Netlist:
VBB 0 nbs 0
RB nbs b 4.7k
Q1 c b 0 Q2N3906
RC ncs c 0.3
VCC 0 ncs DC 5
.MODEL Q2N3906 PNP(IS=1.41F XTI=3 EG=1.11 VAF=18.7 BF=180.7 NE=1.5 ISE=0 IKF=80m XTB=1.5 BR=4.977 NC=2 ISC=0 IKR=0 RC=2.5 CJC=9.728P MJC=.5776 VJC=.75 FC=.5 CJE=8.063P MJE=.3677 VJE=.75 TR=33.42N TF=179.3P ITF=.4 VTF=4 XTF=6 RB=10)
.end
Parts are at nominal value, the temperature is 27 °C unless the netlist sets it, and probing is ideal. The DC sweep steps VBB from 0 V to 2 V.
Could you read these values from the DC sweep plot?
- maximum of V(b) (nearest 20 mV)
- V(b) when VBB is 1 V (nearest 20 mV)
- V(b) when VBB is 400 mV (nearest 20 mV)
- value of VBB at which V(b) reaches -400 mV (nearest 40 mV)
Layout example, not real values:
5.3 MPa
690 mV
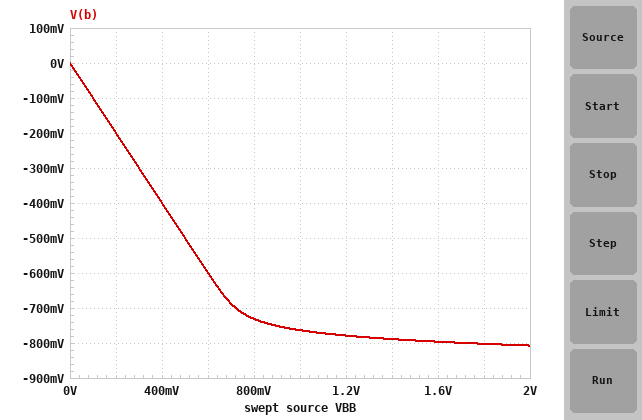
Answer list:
0 V
-760 mV
-400 mV
400 mV
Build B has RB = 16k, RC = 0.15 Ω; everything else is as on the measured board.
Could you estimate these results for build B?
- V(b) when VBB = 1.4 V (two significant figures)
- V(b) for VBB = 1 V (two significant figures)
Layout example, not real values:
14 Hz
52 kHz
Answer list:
-760 mV
-730 mV
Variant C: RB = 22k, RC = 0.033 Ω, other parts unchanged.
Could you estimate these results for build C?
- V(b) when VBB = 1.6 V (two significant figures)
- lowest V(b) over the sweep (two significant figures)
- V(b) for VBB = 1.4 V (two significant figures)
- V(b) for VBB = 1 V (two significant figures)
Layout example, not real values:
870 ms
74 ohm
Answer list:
-760 mV
-770 mV
-750 mV
-730 mV
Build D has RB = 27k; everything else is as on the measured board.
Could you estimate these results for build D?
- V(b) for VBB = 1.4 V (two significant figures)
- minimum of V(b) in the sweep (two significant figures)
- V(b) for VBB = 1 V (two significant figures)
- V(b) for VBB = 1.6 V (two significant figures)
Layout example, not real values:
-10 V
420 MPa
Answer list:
-740 mV
-760 mV
-720 mV
-750 mV
